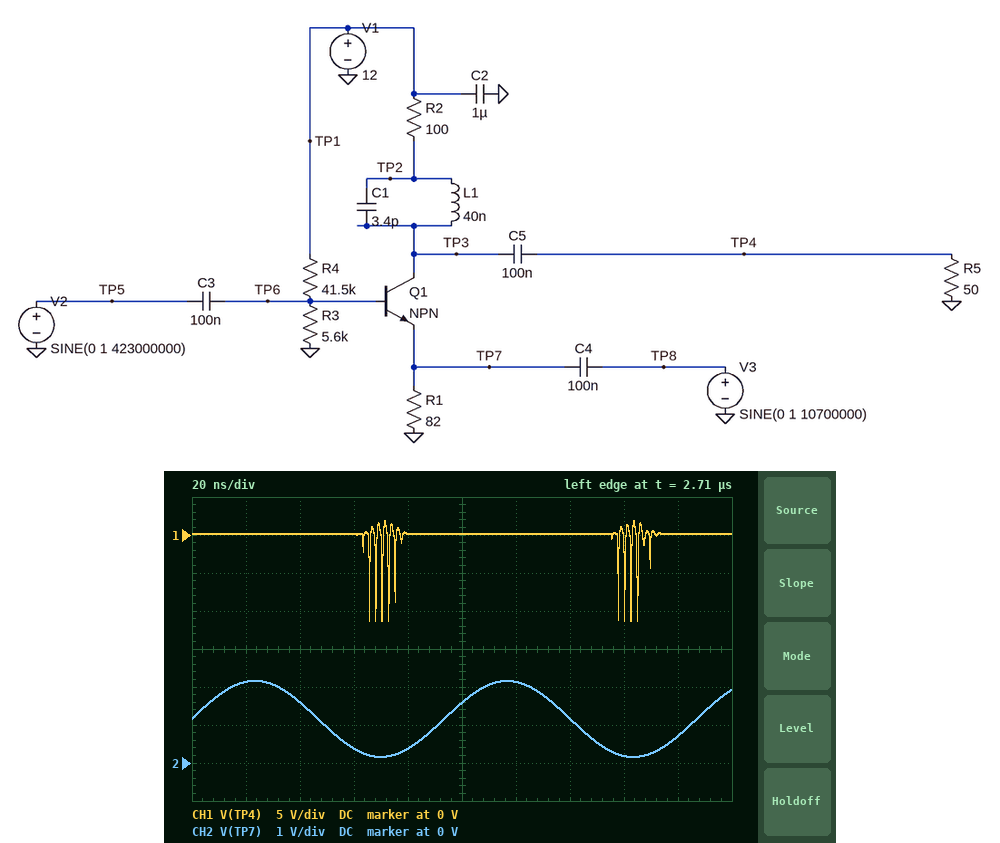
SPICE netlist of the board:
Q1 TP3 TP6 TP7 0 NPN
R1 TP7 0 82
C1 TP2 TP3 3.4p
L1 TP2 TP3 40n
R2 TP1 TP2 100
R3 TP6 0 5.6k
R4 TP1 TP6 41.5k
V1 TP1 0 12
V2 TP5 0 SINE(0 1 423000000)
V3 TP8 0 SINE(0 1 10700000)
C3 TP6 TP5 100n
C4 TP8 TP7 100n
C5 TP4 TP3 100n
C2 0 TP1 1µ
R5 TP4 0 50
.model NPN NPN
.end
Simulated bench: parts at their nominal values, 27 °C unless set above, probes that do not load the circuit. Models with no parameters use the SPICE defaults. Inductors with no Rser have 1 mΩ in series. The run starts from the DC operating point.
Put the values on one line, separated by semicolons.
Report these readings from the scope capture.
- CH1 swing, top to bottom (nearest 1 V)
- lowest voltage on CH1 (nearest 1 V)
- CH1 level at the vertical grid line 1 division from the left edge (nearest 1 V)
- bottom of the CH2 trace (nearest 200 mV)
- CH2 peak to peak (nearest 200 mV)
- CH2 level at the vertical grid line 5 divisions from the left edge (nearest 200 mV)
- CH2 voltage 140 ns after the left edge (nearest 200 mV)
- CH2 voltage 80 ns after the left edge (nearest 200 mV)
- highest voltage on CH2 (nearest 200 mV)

13 V; -11 V; 0 V; 200 mV; 2.0 V; 1.6 V; 1.2 V; 400 mV; 2.2 V
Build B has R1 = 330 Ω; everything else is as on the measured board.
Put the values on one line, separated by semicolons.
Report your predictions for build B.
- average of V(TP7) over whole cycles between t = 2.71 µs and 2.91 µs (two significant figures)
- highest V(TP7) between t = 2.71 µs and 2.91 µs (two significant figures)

1.5 V; 2.5 V
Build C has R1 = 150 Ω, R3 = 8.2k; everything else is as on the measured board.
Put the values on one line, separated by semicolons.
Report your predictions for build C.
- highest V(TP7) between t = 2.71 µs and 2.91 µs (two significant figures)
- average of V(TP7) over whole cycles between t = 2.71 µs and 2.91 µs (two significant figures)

2.6 V; 1.6 V
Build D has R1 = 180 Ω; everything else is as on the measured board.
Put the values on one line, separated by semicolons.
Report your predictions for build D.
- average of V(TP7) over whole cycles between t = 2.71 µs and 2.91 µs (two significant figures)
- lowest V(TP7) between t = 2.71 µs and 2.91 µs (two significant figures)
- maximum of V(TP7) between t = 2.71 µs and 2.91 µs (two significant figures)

1.4 V; 360 mV; 2.4 V
